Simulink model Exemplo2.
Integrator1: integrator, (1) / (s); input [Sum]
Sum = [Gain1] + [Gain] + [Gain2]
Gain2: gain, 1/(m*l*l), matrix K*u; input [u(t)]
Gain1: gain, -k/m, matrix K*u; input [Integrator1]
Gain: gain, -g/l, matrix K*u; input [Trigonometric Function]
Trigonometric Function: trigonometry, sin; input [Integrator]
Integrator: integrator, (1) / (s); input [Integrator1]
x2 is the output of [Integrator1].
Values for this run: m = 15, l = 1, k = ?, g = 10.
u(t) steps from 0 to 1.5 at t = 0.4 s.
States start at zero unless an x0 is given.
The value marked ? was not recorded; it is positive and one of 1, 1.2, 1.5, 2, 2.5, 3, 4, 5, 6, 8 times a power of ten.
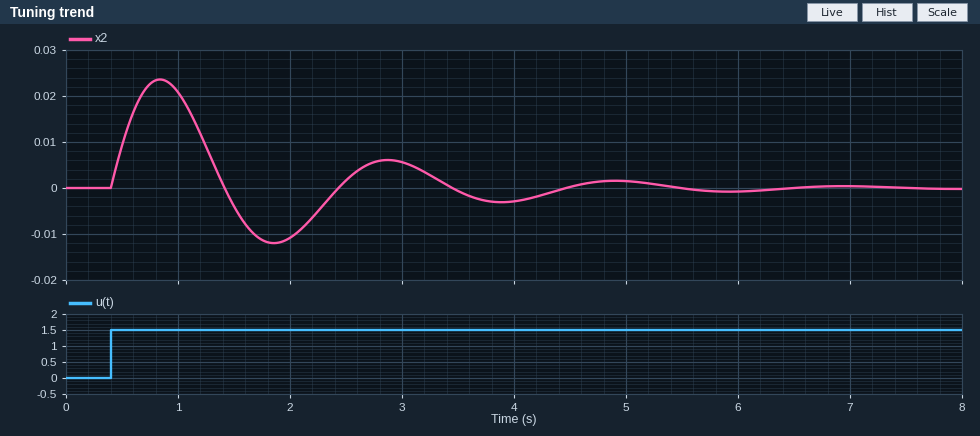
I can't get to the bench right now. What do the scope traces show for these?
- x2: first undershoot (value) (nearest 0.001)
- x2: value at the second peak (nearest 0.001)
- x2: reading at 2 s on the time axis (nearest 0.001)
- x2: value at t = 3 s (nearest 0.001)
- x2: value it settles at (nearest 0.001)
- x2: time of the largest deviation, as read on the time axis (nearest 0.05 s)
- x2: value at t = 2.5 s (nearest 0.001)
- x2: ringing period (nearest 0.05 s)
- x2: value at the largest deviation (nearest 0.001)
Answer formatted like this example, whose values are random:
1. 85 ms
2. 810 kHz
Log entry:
1. -0.012
2. 0.006
3. -0.011
4. 0.006
5. 0.000
6. 0.85 s
7. 0.002
8. 2.05 s
9. 0.024
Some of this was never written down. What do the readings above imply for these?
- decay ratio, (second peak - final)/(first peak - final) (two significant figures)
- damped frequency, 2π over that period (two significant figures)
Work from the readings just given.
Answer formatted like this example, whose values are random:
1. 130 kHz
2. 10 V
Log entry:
1. 0.25
2. 3.1 rad/s
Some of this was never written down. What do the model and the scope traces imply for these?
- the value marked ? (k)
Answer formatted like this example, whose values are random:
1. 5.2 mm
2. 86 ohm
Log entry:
1. 20
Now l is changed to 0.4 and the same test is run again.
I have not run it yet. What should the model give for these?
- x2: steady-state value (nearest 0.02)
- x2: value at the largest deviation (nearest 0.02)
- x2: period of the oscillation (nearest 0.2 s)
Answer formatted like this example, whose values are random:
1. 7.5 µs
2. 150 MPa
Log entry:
1. 0.00
2. 0.10
3. 1.2 s
